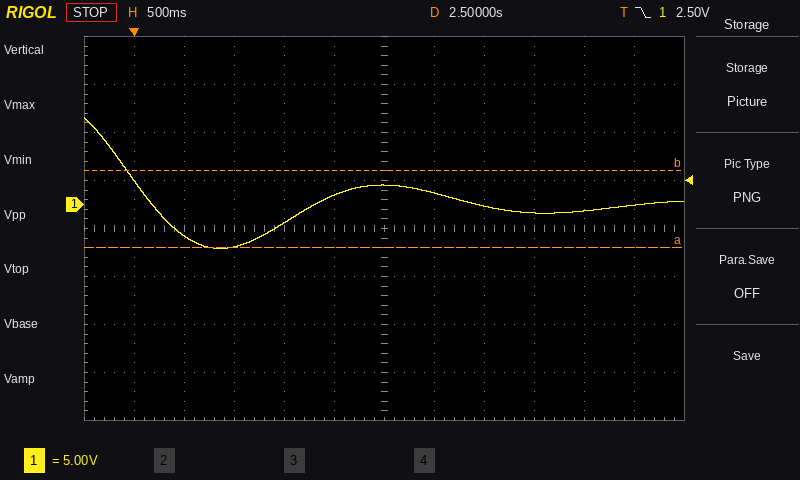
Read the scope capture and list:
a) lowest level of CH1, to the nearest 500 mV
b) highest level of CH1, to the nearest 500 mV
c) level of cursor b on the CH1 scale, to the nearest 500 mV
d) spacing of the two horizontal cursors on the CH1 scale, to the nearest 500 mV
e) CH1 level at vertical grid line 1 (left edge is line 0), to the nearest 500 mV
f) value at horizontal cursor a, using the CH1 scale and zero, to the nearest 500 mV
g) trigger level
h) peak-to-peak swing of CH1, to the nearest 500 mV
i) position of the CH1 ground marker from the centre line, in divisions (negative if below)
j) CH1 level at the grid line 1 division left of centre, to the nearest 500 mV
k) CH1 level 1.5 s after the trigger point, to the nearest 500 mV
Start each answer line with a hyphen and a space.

- -4.5 V
- 9.0 V
- 3.5 V
- 8.0 V
- 2.5 V
- -4.5 V
- 2.50 V
- 13.5 V
- +0.5 div
- 1.0 V
- -2.0 V
